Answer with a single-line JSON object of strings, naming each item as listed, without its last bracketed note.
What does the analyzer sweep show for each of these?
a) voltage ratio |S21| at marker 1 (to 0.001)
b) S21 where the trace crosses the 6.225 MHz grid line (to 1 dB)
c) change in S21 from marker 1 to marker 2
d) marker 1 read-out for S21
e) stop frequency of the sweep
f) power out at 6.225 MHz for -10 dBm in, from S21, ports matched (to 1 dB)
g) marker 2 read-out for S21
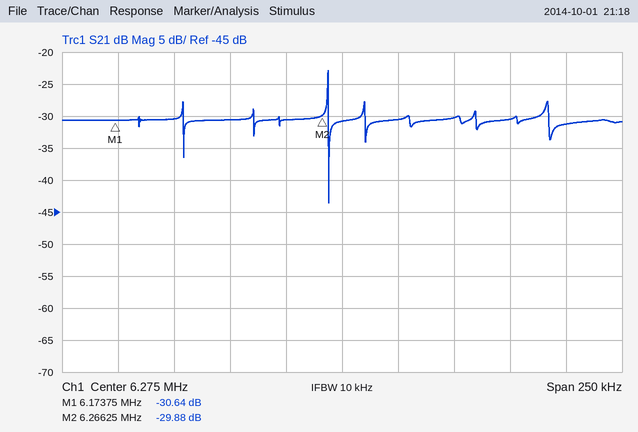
{"voltage ratio |S21| at marker 1": "0.029", "S21 where the trace crosses the 6.225 MHz grid line": "-31 dB", "change in S21 from marker 1 to marker 2": "0.76 dB", "marker 1 read-out for S21": "-30.64 dB", "stop frequency of the sweep": "6.4 MHz", "power out at 6.225 MHz for -10 dBm in, from S21, ports matched": "-41 dBm", "marker 2 read-out for S21": "-29.88 dB"}
